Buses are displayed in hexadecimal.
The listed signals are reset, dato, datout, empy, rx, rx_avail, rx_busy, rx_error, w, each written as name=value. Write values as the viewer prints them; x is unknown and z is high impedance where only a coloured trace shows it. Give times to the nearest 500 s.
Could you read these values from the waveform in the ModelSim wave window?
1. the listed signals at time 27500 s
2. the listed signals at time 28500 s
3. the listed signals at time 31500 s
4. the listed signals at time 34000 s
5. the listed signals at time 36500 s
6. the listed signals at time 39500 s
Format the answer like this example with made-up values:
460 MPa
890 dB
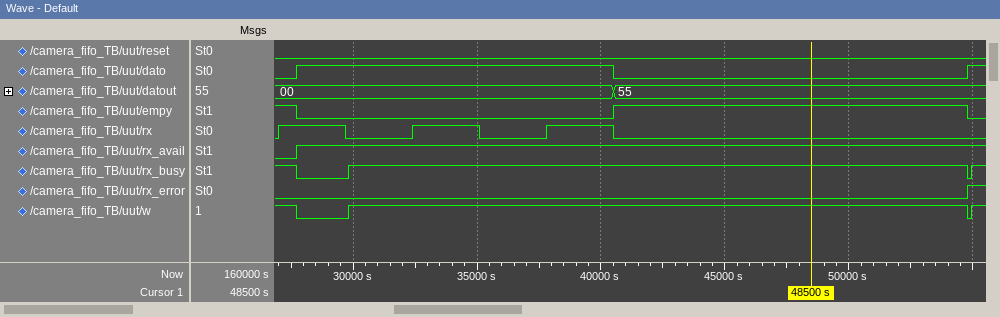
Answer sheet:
reset=0, dato=0, datout=00, empy=1, rx=1, rx_avail=0, rx_busy=1, rx_error=0, w=1
reset=0, dato=1, datout=00, empy=0, rx=1, rx_avail=1, rx_busy=0, rx_error=0, w=0
reset=0, dato=1, datout=00, empy=0, rx=0, rx_avail=1, rx_busy=1, rx_error=0, w=1
reset=0, dato=1, datout=00, empy=0, rx=1, rx_avail=1, rx_busy=1, rx_error=0, w=1
reset=0, dato=1, datout=00, empy=0, rx=0, rx_avail=1, rx_busy=1, rx_error=0, w=1
reset=0, dato=1, datout=00, empy=0, rx=1, rx_avail=1, rx_busy=1, rx_error=0, w=1
